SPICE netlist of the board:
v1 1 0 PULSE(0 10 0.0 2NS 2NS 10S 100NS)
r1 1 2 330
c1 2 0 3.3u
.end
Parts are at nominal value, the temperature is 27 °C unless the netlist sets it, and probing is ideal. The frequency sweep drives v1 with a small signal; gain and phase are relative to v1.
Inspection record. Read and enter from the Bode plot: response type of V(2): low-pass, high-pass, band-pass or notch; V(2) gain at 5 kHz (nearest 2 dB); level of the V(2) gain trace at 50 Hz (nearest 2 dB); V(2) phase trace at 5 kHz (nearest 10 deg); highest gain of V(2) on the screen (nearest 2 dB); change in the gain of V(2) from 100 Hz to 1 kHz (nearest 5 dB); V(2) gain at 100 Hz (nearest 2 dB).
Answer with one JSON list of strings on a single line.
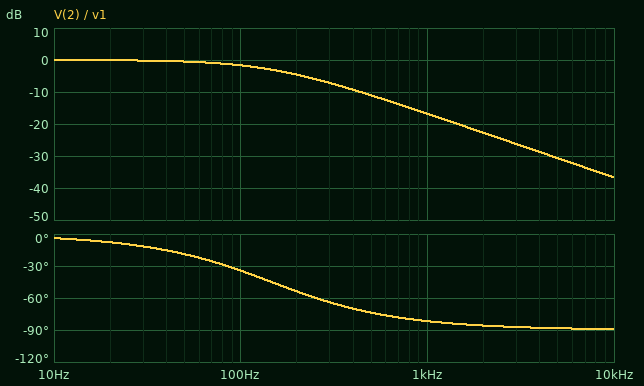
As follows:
["low-pass", "-30 dB", "0 dB", "-90 deg", "0 dB", "-15 dB", "-2 dB"]
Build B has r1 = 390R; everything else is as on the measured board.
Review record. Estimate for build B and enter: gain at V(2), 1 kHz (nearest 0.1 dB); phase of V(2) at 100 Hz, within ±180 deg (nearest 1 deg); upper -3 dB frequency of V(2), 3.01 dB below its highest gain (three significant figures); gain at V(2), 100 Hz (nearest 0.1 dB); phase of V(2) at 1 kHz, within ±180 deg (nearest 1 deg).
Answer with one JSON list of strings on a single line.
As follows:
["-18.2 dB", "-39 deg", "124 Hz", "-2.2 dB", "-83 deg"]
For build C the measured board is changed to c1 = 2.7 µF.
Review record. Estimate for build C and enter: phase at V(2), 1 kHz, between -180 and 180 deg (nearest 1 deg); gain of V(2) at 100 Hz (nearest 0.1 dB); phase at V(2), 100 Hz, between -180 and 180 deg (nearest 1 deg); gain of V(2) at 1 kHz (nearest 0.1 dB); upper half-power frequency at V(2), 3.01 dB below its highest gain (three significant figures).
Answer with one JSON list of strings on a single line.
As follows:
["-80 deg", "-1.2 dB", "-29 deg", "-15.1 dB", "179 Hz"]
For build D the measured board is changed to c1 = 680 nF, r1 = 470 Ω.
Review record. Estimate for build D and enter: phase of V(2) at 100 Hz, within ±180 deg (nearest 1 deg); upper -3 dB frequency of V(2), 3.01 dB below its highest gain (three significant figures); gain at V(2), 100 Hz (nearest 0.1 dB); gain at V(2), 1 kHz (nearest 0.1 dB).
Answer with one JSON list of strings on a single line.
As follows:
["-11 deg", "498 Hz", "-0.2 dB", "-7.0 dB"]
